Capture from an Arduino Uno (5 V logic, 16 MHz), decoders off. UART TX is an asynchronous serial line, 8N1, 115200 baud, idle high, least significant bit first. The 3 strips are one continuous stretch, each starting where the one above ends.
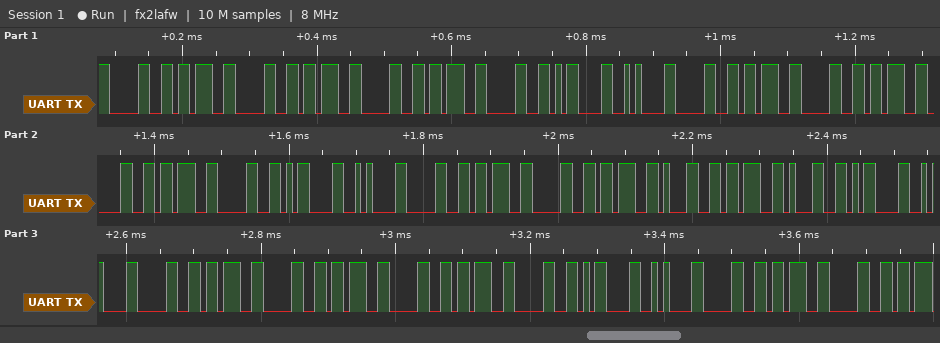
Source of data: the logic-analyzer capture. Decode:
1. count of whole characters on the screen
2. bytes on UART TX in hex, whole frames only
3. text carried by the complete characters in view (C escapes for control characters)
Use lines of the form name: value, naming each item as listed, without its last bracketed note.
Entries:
count of whole characters on the screen: 39
bytes on UART TX in hex, whole frames only: 0x30 0x3B 0x30 0x3B 0x30 0x3B 0x30 0x0D 0x0A 0x30 0x3B 0x30 0x3B 0x30 0x3B 0x30 0x0D 0x0A 0x30 0x3B 0x30 0x3B 0x31 0x3B 0x31 0x0D 0x0A 0x30 0x3B 0x30 0x3B 0x30 0x3B 0x30 0x0D 0x0A 0x30 0x3B 0x30
text carried by the complete characters in view: "0;0;0;0\r\n0;0;0;0\r\n0;0;1;1\r\n0;0;0;0\r\n0;0"
